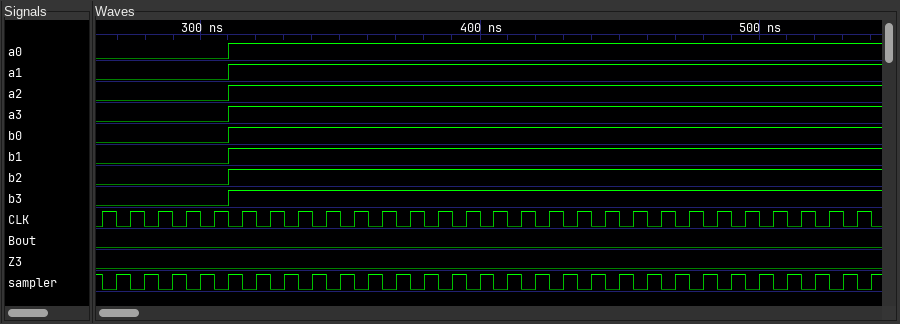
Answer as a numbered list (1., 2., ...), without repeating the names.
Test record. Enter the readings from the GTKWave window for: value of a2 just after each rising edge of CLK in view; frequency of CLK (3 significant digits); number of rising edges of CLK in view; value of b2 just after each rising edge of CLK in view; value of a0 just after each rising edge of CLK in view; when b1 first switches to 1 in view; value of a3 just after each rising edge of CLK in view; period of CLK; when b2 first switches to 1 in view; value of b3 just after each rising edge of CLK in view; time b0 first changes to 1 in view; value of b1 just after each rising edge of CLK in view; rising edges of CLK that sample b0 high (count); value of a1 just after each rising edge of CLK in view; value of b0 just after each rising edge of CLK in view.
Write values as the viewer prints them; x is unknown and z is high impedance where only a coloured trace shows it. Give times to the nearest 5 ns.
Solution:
1. 0 0 0 0 0 1 1 1 1 1 1 1 1 1 1 1 1 1 1 1 1 1 1 1 1 1 1 1
2. 100 MHz
3. 28
4. 0 0 0 0 0 1 1 1 1 1 1 1 1 1 1 1 1 1 1 1 1 1 1 1 1 1 1 1
5. 0 0 0 0 0 1 1 1 1 1 1 1 1 1 1 1 1 1 1 1 1 1 1 1 1 1 1 1
6. 310 ns
7. 0 0 0 0 0 1 1 1 1 1 1 1 1 1 1 1 1 1 1 1 1 1 1 1 1 1 1 1
8. 10 ns
9. 310 ns
10. 0 0 0 0 0 1 1 1 1 1 1 1 1 1 1 1 1 1 1 1 1 1 1 1 1 1 1 1
11. 310 ns
12. 0 0 0 0 0 1 1 1 1 1 1 1 1 1 1 1 1 1 1 1 1 1 1 1 1 1 1 1
13. 23
14. 0 0 0 0 0 1 1 1 1 1 1 1 1 1 1 1 1 1 1 1 1 1 1 1 1 1 1 1
15. 0 0 0 0 0 1 1 1 1 1 1 1 1 1 1 1 1 1 1 1 1 1 1 1 1 1 1 1
